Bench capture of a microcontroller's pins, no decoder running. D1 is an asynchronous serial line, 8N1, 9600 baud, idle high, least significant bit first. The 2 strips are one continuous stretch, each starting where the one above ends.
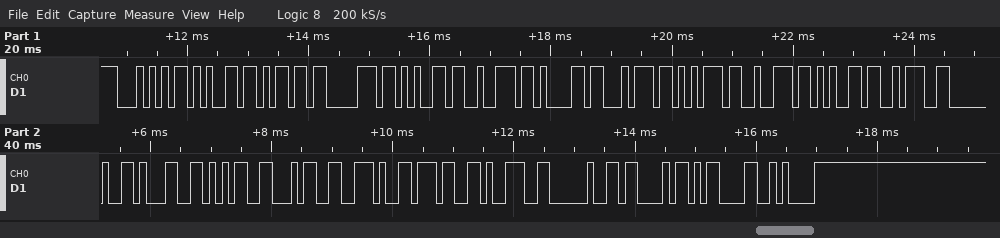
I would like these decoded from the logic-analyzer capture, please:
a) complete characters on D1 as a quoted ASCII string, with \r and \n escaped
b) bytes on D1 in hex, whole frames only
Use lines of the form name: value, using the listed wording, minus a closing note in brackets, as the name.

complete characters on D1 as a quoted ASCII string, with \r and \n escaped: "Temperature: 154.79 C\r\n"
bytes on D1 in hex, whole frames only: 0x54 0x65 0x6D 0x70 0x65 0x72 0x61 0x74 0x75 0x72 0x65 0x3A 0x20 0x31 0x35 0x34 0x2E 0x37 0x39 0x20 0x43 0x0D 0x0A
